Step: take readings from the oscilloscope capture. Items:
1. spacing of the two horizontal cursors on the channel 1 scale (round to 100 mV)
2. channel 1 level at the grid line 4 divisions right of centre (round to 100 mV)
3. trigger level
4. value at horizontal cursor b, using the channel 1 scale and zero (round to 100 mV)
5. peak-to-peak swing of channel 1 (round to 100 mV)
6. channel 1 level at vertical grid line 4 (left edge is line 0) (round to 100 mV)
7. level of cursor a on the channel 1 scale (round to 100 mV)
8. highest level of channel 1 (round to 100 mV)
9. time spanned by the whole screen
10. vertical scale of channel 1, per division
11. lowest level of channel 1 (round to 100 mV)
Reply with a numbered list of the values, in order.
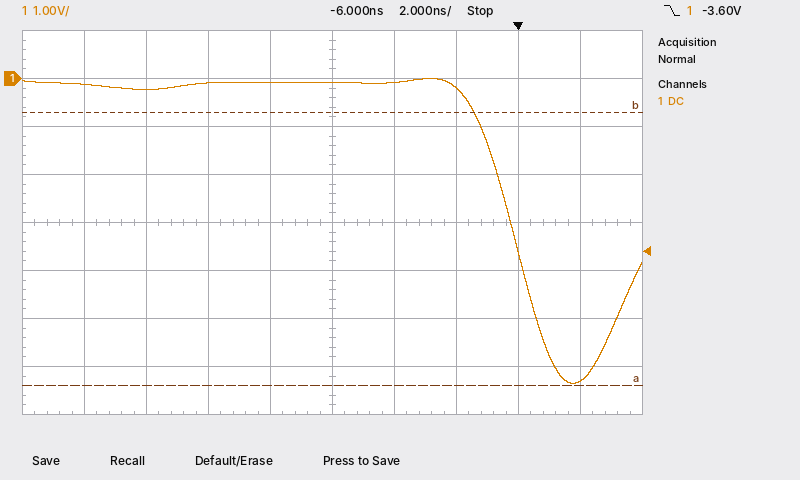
1. 5.7 V
2. -6.3 V
3. -3.60 V
4. -700 mV
5. 6.4 V
6. -100 mV
7. -6.4 V
8. 0.0 V
9. 20 ns
10. 1 V
11. -6.4 V
